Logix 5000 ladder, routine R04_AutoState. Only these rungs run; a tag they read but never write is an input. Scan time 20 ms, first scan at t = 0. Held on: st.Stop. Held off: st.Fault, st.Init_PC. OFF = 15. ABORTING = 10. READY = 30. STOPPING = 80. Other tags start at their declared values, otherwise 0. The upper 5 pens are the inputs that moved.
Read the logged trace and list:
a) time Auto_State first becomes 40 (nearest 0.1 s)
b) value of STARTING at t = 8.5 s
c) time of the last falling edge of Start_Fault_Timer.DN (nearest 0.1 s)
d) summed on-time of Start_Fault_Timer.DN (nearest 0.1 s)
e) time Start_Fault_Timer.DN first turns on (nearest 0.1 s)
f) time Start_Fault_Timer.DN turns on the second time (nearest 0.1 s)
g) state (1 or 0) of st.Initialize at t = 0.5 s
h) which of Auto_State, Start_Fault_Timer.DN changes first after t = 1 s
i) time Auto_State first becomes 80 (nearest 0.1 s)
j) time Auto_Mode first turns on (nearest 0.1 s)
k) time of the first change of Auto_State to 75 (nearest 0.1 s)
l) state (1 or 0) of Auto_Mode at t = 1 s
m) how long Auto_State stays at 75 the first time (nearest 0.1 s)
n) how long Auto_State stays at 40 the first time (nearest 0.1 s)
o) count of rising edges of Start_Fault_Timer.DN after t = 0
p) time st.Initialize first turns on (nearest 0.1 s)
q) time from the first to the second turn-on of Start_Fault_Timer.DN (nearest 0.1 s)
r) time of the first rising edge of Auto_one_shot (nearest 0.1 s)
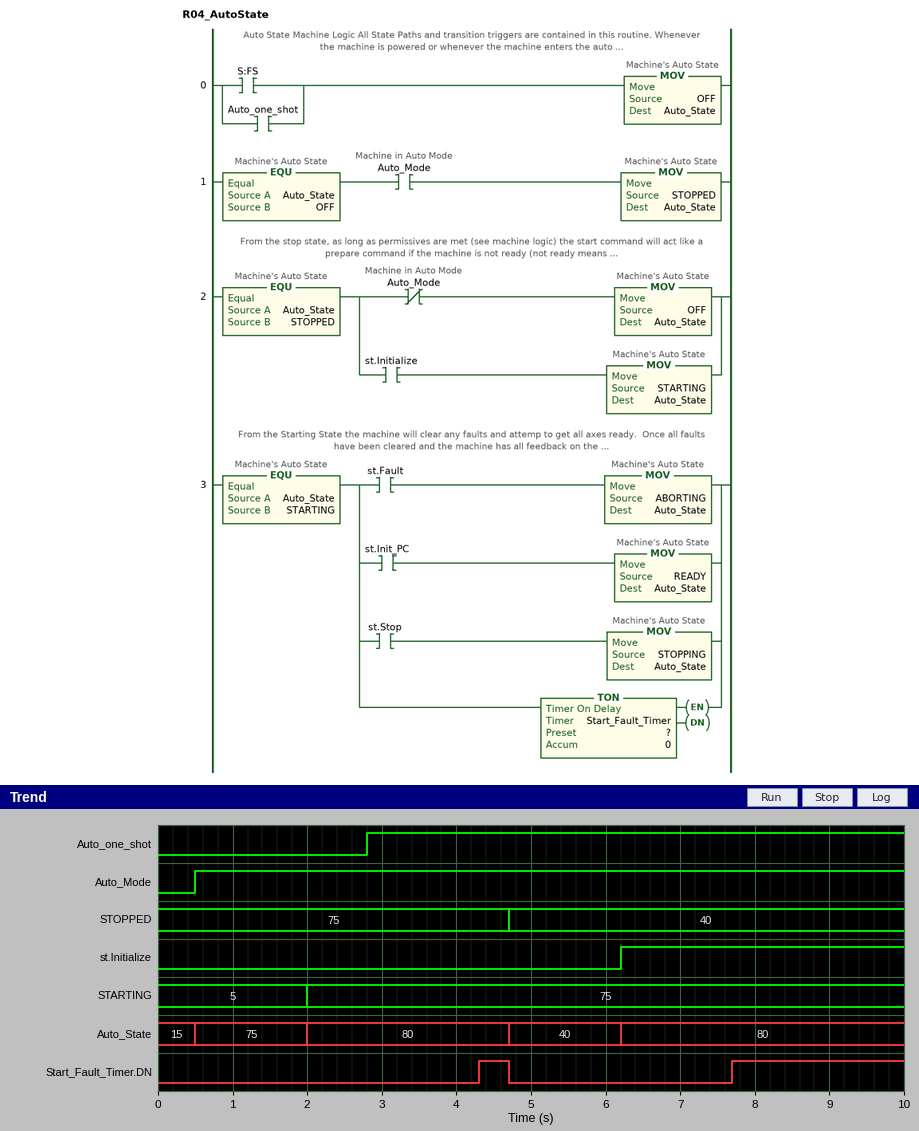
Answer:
4.7 s
75
4.7 s
2.7 s
4.3 s
7.7 s
0
Auto_State
2.0 s
0.5 s
0.5 s
1
1.5 s
1.5 s
2
6.2 s
3.4 s
2.8 s
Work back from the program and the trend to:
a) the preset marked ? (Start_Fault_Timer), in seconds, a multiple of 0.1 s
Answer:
1.5 s
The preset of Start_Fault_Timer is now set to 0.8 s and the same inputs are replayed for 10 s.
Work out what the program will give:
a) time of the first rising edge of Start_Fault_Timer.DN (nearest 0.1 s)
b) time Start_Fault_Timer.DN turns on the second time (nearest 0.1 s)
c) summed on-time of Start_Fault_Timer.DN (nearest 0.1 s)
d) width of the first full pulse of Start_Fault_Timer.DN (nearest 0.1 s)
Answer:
3.6 s
7.0 s
4.1 s
1.1 s
